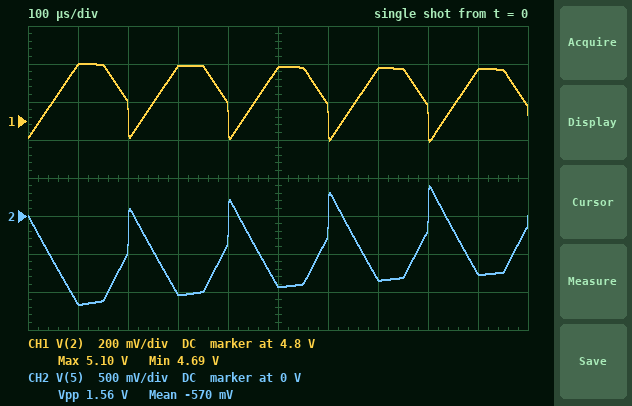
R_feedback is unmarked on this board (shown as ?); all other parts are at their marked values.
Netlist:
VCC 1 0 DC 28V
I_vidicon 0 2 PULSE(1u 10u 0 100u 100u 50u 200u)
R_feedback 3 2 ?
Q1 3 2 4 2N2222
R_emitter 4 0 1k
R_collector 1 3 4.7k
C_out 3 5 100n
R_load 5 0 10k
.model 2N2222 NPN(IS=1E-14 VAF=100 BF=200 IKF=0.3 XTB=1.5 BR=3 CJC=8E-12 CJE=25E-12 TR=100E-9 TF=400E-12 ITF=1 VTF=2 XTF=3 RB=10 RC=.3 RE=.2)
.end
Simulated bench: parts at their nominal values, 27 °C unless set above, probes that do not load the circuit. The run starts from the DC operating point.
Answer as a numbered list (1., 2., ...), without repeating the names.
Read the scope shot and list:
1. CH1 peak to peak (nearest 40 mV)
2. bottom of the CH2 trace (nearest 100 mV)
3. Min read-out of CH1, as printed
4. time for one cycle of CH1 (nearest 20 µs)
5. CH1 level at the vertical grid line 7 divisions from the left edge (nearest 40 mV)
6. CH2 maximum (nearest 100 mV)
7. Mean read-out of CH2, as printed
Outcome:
1. 400 mV
2. -1.2 V
3. 4.69 V
4. 200 µs
5. 5.08 V
6. 400 mV
7. -570 mV
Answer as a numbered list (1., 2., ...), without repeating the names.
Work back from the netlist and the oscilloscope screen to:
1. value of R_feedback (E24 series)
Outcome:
1. 240 kΩ
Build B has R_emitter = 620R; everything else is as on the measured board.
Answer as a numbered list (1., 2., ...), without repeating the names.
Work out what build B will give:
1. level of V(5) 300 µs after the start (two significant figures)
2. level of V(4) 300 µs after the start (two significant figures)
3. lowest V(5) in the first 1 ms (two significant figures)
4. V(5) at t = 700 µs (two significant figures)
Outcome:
1. -1.1 V
2. 2.9 V
3. -1.3 V
4. -900 mV
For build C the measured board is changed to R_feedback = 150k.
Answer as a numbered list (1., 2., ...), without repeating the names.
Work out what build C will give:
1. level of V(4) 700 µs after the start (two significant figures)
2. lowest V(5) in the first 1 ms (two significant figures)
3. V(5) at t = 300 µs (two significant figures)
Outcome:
1. 4.5 V
2. -800 mV
3. -710 mV
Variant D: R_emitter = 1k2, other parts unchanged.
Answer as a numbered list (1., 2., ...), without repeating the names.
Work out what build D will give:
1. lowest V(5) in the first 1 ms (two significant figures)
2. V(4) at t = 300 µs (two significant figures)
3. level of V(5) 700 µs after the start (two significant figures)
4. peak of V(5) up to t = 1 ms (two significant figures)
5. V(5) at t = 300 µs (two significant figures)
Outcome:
1. -1.1 V
2. 5.1 V
3. -810 mV
4. 370 mV
5. -1.0 V
